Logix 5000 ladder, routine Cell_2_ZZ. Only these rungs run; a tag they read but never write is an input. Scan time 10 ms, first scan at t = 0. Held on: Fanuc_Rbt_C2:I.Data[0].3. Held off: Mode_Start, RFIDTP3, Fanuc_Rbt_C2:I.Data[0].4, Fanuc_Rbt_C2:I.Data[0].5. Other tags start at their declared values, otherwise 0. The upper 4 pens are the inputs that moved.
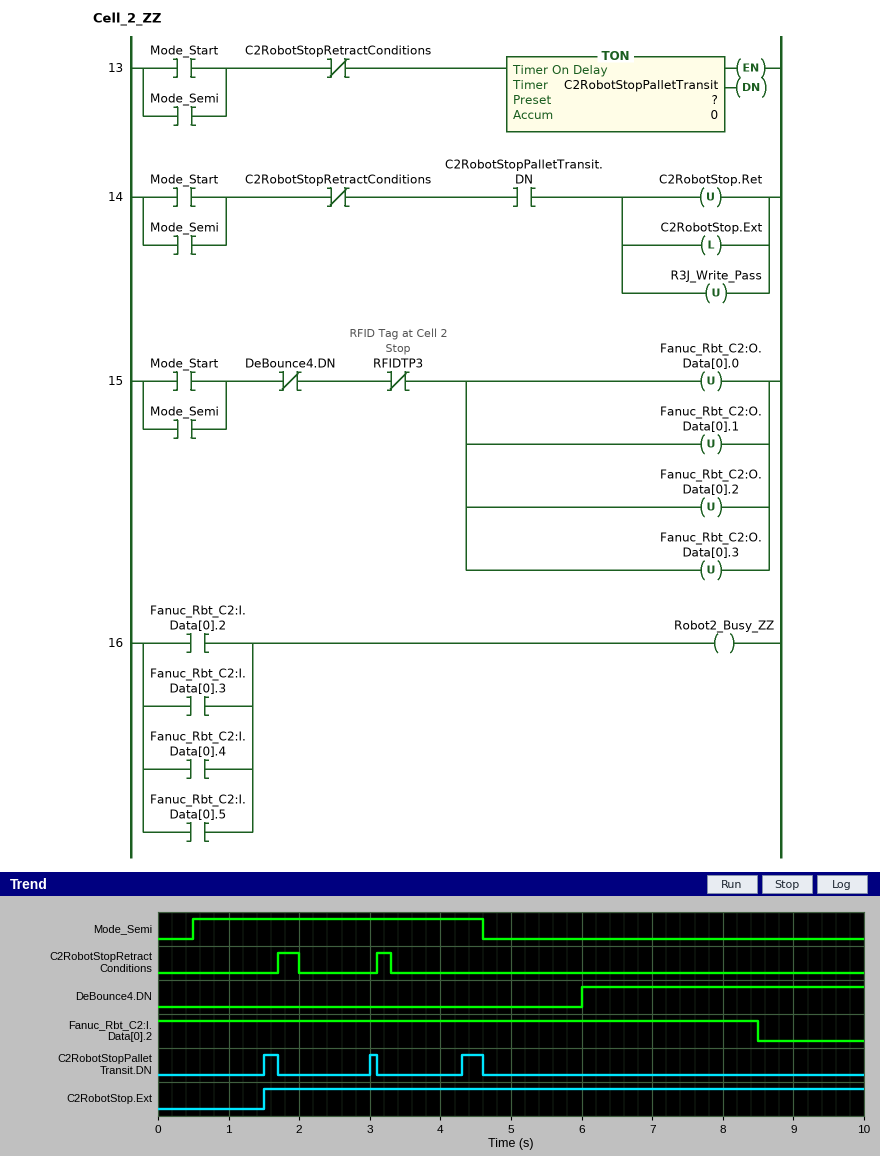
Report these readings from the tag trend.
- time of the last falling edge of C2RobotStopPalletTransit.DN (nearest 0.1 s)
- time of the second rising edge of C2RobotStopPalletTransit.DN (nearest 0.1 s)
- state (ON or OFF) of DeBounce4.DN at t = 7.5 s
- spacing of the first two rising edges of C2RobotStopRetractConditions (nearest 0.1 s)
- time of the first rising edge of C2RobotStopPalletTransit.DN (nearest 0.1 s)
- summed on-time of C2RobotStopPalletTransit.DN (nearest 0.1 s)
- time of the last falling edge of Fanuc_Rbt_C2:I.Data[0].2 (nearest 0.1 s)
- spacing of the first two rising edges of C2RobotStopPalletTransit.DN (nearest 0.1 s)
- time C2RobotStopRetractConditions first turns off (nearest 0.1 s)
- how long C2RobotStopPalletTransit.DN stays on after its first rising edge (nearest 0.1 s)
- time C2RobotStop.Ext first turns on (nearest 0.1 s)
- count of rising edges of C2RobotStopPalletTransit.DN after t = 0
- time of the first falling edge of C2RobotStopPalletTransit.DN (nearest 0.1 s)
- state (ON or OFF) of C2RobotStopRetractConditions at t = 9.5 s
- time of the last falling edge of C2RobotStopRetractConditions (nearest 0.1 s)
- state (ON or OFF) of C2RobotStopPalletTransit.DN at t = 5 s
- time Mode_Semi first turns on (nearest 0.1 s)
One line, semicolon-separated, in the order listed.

4.6 s; 3.0 s; ON; 1.4 s; 1.5 s; 0.6 s; 8.5 s; 1.5 s; 2.0 s; 0.2 s; 1.5 s; 3; 1.7 s; OFF; 3.3 s; OFF; 0.5 s
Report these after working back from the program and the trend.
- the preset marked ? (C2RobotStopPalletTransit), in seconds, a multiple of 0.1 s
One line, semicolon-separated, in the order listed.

1.0 s
